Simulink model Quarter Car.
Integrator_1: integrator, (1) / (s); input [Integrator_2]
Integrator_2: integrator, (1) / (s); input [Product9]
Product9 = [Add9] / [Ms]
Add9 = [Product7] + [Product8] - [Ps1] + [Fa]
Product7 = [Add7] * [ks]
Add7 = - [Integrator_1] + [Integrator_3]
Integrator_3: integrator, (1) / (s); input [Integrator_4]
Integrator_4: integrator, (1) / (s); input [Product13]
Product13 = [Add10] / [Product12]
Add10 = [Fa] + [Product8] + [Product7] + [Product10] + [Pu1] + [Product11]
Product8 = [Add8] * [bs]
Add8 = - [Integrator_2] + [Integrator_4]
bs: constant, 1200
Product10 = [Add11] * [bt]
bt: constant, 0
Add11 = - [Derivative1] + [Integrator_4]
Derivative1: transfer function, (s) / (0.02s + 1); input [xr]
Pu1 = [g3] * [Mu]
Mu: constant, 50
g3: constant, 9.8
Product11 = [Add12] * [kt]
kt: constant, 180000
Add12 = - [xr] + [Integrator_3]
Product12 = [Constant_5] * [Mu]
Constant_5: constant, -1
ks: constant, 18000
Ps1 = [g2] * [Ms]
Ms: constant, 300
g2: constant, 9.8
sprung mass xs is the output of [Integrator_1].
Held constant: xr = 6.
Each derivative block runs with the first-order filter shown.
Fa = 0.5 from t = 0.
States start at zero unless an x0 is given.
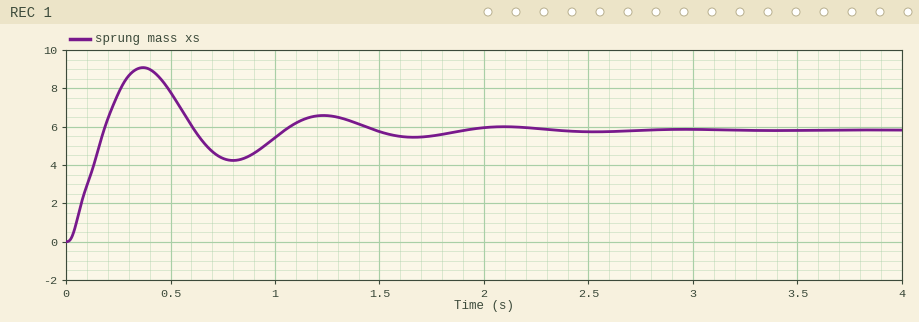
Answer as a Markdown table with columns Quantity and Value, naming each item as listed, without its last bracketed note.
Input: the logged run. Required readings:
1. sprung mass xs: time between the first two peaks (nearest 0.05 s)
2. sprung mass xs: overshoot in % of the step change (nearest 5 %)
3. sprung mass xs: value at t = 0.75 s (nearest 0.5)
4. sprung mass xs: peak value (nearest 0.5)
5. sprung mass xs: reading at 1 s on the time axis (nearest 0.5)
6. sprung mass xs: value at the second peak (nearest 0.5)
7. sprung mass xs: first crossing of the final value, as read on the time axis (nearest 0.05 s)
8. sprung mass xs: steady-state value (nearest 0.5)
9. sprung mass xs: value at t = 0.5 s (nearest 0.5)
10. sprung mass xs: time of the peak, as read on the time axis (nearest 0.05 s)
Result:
| Quantity | Value |
|---|---|
| sprung mass xs: time between the first two peaks | 0.85 s |
| sprung mass xs: overshoot in % of the step change | 55 % |
| sprung mass xs: value at t = 0.75 s | 4.5 |
| sprung mass xs: peak value | 9.0 |
| sprung mass xs: reading at 1 s on the time axis | 5.5 |
| sprung mass xs: value at the second peak | 6.5 |
| sprung mass xs: first crossing of the final value, as read on the time axis | 0.20 s |
| sprung mass xs: steady-state value | 6.0 |
| sprung mass xs: value at t = 0.5 s | 8.0 |
| sprung mass xs: time of the peak, as read on the time axis | 0.35 s |
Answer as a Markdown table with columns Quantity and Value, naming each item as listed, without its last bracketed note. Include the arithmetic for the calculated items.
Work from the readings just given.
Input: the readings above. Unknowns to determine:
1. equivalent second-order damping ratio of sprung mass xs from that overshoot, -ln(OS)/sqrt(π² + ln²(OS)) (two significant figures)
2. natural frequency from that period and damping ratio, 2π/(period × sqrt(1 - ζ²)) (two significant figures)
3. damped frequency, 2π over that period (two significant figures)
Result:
| Quantity | Value |
|---|---|
| equivalent second-order damping ratio of sprung mass xs from that overshoot, -ln(OS)/sqrt(π² + ln²(OS)) | ln(0.55) = -0.598; 0.598 / sqrt(9.870 + 0.357) = 0.19 |
| natural frequency from that period and damping ratio, 2π/(period × sqrt(1 - ζ²)) | 2π / (0.85 × sqrt(1 - 0.19²)) = 7.5 rad/s |
| damped frequency, 2π over that period | 2π / 0.85 = 7.4 rad/s |
